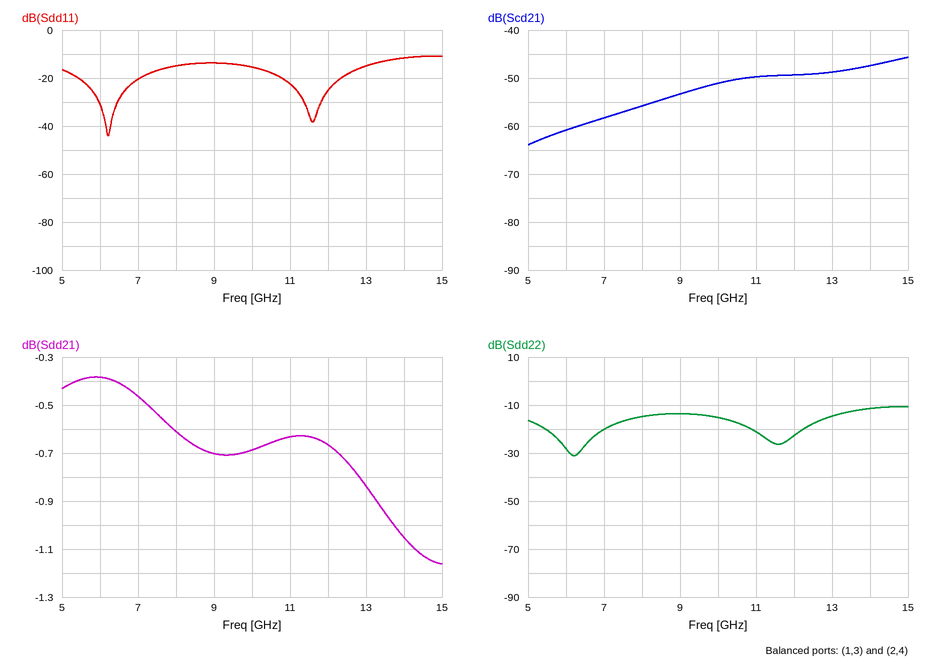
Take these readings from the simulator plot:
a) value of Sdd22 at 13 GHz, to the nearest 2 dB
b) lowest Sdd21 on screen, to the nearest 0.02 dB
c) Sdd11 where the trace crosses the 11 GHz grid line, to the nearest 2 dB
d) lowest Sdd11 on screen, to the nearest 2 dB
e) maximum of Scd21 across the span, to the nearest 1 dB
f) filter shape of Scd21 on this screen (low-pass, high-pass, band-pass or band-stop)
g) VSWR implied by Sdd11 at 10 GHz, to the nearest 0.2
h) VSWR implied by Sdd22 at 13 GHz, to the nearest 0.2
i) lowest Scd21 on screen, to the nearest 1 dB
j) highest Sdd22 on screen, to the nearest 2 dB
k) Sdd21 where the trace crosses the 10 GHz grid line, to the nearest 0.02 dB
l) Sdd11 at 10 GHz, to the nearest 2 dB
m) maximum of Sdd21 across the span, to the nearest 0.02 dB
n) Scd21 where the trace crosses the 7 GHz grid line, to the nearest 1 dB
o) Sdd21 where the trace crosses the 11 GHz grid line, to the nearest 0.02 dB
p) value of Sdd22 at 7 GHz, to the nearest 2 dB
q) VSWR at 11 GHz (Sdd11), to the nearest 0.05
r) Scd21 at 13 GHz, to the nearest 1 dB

-14 dB
-1.16 dB
-22 dB
-44 dB
-46 dB
high-pass
1.4
1.4
-64 dB
-10 dB
-0.68 dB
-16 dB
-0.38 dB
-58 dB
-0.64 dB
-20 dB
1.15
-49 dB
